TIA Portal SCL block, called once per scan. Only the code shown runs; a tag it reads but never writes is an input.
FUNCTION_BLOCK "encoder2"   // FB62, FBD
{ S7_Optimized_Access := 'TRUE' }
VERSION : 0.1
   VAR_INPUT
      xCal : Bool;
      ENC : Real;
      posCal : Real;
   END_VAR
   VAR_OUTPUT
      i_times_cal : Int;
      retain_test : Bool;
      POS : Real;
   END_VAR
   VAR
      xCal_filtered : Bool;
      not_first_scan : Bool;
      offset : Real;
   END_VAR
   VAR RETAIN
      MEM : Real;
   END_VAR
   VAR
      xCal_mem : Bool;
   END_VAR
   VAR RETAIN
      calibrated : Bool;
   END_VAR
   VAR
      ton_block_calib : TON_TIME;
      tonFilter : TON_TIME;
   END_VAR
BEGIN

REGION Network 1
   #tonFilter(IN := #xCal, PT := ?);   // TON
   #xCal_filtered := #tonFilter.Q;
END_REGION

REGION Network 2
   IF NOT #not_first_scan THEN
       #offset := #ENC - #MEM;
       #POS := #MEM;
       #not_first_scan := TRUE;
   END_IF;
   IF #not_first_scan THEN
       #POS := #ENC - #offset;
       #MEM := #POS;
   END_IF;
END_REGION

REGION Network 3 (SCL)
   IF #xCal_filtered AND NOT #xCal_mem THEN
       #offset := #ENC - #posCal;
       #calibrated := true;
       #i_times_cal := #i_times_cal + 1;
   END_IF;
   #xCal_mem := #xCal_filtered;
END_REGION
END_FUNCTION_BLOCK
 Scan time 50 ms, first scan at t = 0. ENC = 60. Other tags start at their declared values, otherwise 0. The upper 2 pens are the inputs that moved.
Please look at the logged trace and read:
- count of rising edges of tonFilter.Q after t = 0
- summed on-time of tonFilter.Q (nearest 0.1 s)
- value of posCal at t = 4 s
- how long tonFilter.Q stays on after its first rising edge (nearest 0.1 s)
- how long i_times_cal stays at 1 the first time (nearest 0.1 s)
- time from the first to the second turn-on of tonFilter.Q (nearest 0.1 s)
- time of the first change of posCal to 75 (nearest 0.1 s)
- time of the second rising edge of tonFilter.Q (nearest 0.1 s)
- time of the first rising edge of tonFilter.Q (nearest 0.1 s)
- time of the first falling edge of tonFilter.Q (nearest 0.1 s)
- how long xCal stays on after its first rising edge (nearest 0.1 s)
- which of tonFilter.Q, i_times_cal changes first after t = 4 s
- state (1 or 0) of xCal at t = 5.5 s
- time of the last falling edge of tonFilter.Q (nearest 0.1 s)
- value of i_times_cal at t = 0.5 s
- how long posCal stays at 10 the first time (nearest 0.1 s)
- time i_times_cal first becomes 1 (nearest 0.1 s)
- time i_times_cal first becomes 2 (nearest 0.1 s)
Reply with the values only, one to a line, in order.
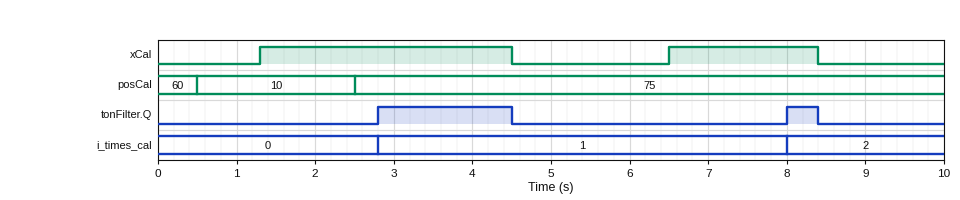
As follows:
2
2.1 s
75
1.7 s
5.2 s
5.2 s
2.5 s
8.0 s
2.8 s
4.5 s
3.2 s
tonFilter.Q
0
8.4 s
0
2.0 s
2.8 s
8.0 s
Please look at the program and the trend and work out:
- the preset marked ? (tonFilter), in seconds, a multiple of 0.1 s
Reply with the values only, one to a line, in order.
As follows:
1.5 s
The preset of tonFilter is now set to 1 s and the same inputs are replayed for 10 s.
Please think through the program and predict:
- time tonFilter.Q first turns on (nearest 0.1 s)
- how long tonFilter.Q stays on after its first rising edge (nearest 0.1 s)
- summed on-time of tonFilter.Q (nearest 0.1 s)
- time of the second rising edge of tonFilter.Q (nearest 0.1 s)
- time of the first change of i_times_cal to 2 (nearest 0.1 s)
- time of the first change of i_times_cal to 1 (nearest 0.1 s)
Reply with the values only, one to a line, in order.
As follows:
2.3 s
2.2 s
3.1 s
7.5 s
7.5 s
2.3 s
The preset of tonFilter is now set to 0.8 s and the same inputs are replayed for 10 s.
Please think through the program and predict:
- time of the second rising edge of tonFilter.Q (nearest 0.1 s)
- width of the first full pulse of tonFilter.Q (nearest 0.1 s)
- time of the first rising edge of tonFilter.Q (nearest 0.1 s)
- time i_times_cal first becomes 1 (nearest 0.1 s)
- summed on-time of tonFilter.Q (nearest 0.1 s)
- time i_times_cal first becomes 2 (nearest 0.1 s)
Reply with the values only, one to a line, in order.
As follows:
7.3 s
2.4 s
2.1 s
2.1 s
3.5 s
7.3 s
